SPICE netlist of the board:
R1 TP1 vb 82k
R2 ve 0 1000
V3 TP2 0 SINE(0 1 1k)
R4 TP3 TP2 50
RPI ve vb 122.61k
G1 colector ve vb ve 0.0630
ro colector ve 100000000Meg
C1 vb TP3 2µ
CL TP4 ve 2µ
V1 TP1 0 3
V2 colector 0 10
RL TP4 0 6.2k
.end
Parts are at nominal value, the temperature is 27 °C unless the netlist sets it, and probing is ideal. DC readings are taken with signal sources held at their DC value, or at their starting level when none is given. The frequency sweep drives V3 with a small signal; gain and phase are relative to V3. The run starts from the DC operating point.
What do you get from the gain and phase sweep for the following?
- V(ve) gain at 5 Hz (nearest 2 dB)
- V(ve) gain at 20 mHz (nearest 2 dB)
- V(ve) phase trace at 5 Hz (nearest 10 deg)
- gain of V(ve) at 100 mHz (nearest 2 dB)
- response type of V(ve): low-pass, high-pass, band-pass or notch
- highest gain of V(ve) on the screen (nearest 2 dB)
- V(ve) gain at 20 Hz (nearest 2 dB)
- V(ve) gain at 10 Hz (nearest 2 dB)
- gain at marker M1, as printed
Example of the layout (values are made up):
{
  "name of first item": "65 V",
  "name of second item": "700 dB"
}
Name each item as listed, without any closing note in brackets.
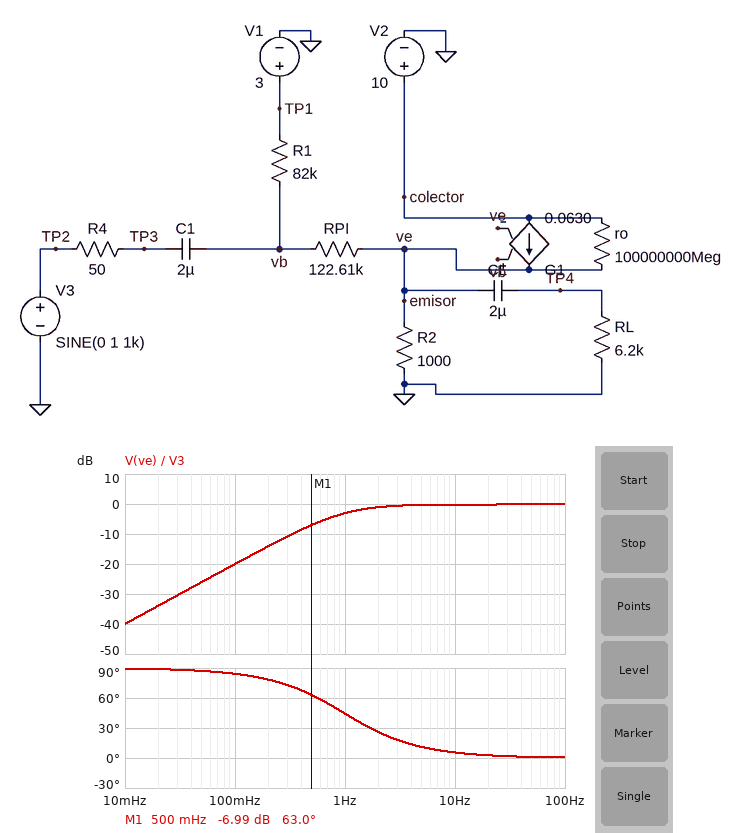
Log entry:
{
  "V(ve) gain at 5 Hz": "0 dB",
  "V(ve) gain at 20 mHz": "-34 dB",
  "V(ve) phase trace at 5 Hz": "10 deg",
  "gain of V(ve) at 100 mHz": "-20 dB",
  "response type of V(ve): low-pass, high-pass, band-pass or notch": "high-pass",
  "highest gain of V(ve) on the screen": "0 dB",
  "V(ve) gain at 20 Hz": "0 dB",
  "V(ve) gain at 10 Hz": "0 dB",
  "gain at marker M1, as printed": "-6.99 dB"
}
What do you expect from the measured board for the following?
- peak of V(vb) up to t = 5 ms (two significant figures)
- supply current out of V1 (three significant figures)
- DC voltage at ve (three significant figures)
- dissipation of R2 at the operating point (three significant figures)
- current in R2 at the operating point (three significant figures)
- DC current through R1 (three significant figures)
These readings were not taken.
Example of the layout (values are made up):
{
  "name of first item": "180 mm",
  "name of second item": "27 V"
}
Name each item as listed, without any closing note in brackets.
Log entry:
{
  "peak of V(vb) up to t = 5 ms": "4.0 V",
  "supply current out of V1": "378 nA",
  "DC voltage at ve": "2.92 V",
  "dissipation of R2 at the operating point": "8.54 mW",
  "current in R2 at the operating point": "2.92 mA",
  "DC current through R1": "378 nA"
}
